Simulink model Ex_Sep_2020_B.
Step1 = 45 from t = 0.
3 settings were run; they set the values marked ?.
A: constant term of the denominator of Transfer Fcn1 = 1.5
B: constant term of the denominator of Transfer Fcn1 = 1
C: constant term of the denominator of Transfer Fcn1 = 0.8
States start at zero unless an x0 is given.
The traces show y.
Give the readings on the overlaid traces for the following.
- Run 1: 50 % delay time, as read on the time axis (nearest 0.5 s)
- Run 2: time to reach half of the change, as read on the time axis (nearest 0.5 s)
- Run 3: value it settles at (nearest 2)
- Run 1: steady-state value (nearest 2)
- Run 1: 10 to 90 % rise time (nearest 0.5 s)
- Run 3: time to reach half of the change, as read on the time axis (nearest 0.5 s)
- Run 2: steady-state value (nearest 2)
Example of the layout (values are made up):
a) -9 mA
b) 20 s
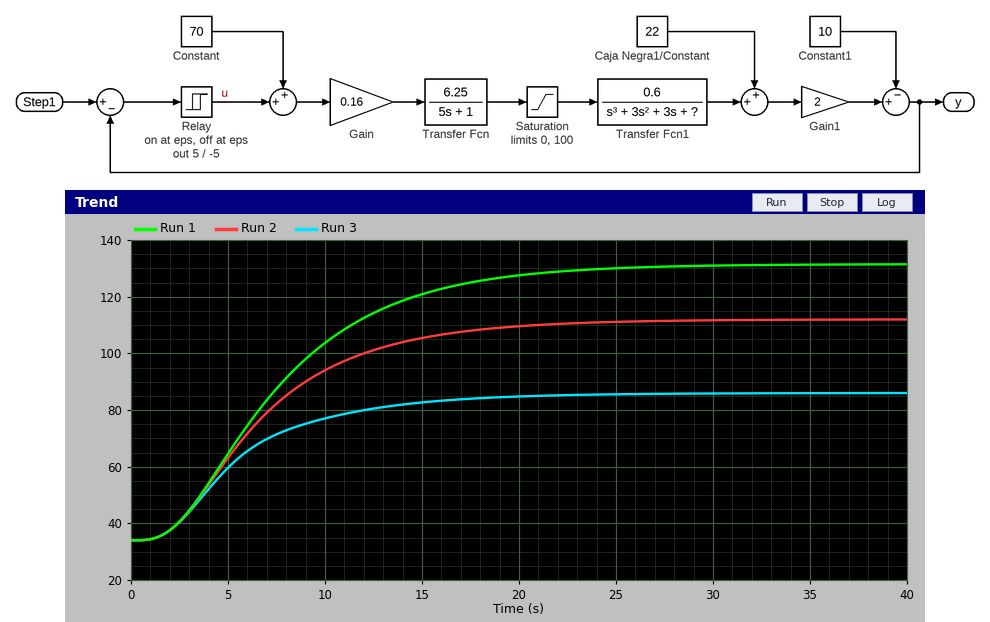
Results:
a) 7.0 s
b) 6.0 s
c) 86
d) 132
e) 12.5 s
f) 5.0 s
g) 112
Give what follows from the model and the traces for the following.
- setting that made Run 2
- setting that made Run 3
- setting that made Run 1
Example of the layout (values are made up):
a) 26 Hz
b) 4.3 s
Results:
a) B
b) A
c) C
